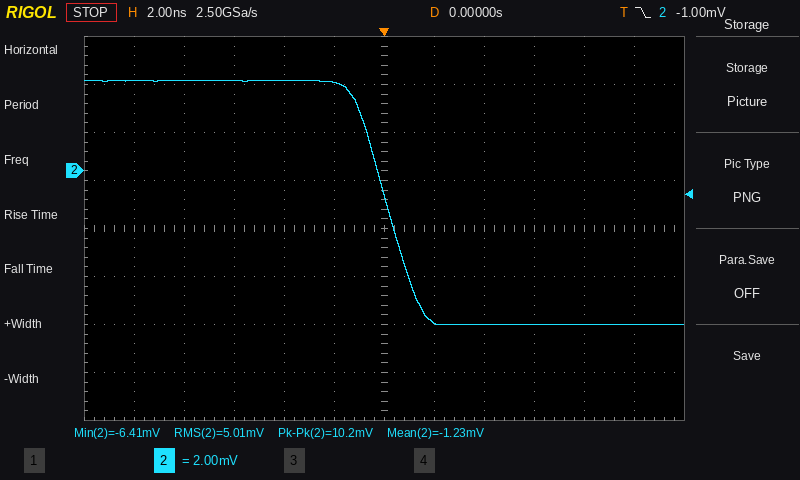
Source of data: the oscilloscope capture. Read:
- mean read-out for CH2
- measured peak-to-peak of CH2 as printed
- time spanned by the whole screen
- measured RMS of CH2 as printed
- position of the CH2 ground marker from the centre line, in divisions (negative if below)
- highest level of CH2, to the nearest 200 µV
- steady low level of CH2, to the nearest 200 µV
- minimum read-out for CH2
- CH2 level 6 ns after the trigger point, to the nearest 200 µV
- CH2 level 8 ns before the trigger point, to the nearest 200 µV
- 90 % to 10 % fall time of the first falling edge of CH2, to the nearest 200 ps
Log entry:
-1.23 mV
10.2 mV
24 ns
5.01 mV
+1.2 div
3.8 mV
-6.4 mV
-6.41 mV
-6.4 mV
3.8 mV
2.4 ns
